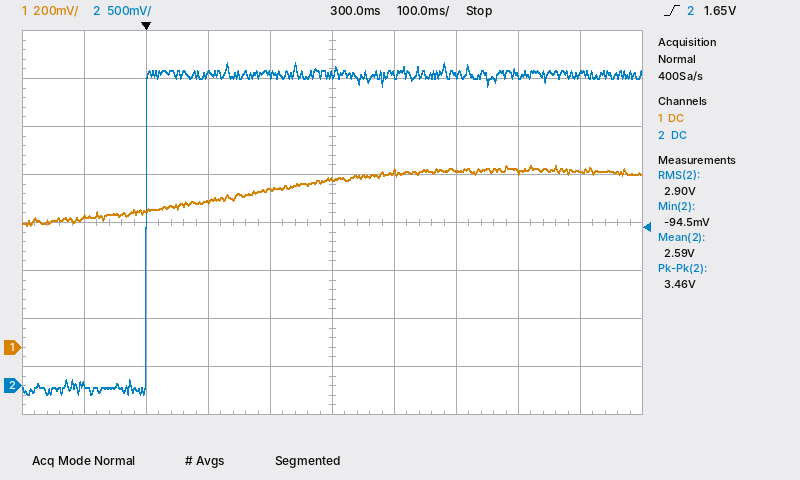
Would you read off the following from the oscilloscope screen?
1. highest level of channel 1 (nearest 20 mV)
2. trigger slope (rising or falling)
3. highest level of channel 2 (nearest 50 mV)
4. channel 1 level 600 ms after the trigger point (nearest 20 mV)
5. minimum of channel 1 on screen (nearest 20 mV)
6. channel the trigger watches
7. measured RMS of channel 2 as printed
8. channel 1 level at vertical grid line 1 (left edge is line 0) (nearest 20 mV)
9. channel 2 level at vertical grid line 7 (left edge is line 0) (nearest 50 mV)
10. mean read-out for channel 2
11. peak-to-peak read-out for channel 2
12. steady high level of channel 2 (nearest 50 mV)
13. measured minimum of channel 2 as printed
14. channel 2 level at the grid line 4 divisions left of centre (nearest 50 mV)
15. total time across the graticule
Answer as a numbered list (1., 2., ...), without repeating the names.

1. 760 mV
2. rising
3. 3.35 V
4. 740 mV
5. 500 mV
6. channel 2
7. 2.90 V
8. 540 mV
9. 3.25 V
10. 2.59 V
11. 3.46 V
12. 3.25 V
13. -94.5 mV
14. 0 mV
15. 1 s
